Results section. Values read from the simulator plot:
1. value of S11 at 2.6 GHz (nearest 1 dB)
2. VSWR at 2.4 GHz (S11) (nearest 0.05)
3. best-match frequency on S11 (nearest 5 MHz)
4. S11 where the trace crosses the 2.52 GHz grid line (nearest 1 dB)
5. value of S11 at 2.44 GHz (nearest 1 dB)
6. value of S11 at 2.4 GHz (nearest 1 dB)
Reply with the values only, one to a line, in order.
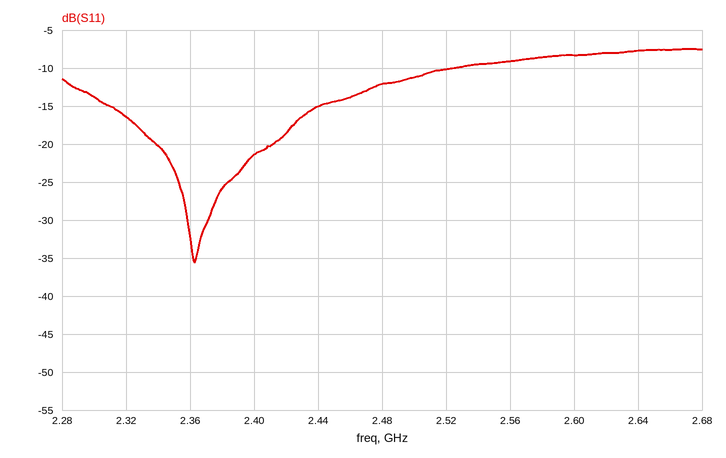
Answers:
-8 dB
1.20
2.365 GHz
-10 dB
-15 dB
-21 dB
